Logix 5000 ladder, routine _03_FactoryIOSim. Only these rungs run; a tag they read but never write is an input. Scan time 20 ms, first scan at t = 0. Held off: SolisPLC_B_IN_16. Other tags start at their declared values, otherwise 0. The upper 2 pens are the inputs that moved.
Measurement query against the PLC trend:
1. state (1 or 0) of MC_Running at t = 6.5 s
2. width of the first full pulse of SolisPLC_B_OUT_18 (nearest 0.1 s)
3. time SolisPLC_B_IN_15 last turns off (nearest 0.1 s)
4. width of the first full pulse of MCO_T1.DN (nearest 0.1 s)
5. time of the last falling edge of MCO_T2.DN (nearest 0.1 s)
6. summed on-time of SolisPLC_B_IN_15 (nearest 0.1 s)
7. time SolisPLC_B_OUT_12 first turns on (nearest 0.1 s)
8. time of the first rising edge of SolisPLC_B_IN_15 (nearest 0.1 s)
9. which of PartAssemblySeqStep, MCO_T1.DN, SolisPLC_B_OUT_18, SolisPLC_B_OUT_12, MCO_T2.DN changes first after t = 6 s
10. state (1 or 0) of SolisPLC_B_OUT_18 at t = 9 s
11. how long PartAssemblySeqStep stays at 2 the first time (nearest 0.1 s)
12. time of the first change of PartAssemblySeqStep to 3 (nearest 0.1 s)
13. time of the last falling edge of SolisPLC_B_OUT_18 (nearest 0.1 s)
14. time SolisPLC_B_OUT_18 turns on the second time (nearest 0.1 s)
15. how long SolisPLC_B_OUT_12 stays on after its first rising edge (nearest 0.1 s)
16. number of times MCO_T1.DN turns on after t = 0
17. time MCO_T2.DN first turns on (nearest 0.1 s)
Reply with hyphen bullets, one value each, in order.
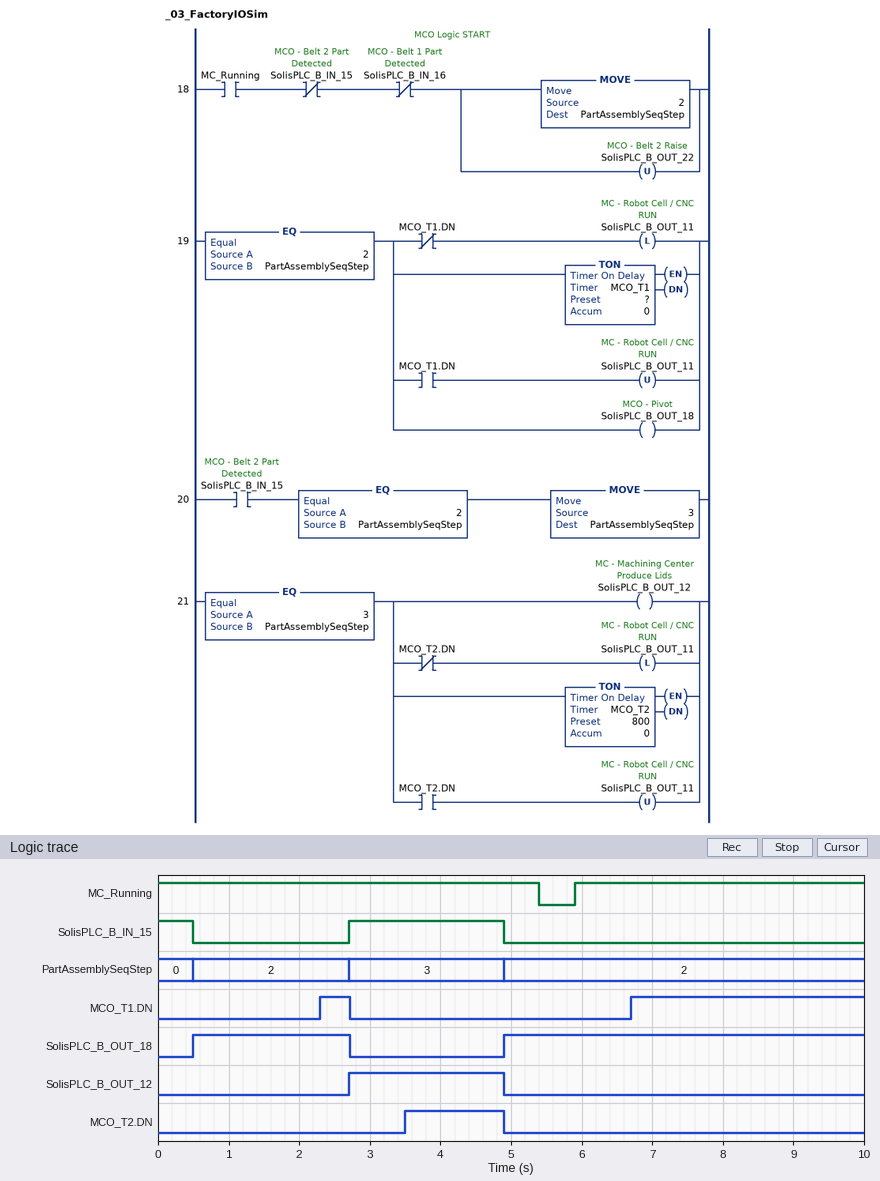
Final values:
- 1
- 2.2 s
- 4.9 s
- 0.4 s
- 4.9 s
- 2.7 s
- 2.7 s
- 2.7 s
- MCO_T1.DN
- 1
- 2.2 s
- 2.7 s
- 2.7 s
- 4.9 s
- 2.2 s
- 2
- 3.5 s
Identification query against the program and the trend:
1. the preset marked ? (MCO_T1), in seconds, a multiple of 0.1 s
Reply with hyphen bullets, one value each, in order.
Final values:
- 1.8 s
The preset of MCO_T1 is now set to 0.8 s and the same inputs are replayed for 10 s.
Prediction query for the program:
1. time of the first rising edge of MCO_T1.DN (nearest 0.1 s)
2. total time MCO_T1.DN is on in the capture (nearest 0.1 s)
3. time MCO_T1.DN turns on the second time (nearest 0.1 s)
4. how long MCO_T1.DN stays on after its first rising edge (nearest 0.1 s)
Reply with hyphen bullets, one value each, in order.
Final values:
- 1.3 s
- 5.7 s
- 5.7 s
- 1.4 s
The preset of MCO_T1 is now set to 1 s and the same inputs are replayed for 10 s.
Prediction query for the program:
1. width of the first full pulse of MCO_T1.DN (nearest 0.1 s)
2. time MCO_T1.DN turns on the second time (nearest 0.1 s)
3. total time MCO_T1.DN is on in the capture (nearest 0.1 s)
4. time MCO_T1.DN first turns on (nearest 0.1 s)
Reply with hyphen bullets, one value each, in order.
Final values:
- 1.2 s
- 5.9 s
- 5.3 s
- 1.5 s
